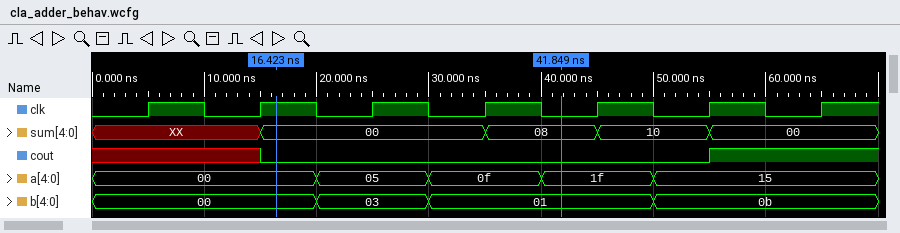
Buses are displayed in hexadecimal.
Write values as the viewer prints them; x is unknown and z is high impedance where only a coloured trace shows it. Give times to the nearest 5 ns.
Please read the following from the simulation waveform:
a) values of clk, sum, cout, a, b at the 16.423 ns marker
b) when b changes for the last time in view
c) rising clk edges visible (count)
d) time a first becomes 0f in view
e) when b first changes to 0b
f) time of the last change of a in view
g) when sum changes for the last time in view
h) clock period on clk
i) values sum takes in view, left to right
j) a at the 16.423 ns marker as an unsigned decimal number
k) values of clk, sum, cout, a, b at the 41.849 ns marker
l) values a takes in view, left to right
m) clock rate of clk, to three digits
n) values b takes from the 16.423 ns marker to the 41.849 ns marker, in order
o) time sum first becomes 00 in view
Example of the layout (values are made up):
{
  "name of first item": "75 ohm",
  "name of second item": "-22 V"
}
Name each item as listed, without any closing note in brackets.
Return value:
{
  "values of clk, sum, cout, a, b at the 16.423 ns marker": "clk=1, sum=00, cout=0, a=00, b=00",
  "when b changes for the last time in view": "50 ns",
  "rising clk edges visible": "7",
  "time a first becomes 0f in view": "30 ns",
  "when b first changes to 0b": "50 ns",
  "time of the last change of a in view": "50 ns",
  "when sum changes for the last time in view": "55 ns",
  "clock period on clk": "10 ns",
  "values sum takes in view, left to right": "XX, 00, 08, 10, 00",
  "a at the 16.423 ns marker as an unsigned decimal number": "0",
  "values of clk, sum, cout, a, b at the 41.849 ns marker": "clk=0, sum=08, cout=0, a=1f, b=01",
  "values a takes in view, left to right": "00, 05, 0f, 1f, 15",
  "clock rate of clk, to three digits": "100 MHz",
  "values b takes from the 16.423 ns marker to the 41.849 ns marker, in order": "00, 03, 01",
  "time sum first becomes 00 in view": "15 ns"
}
